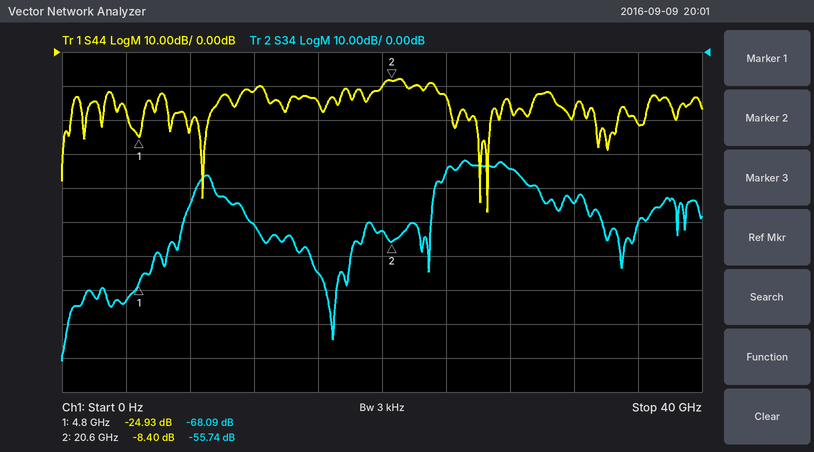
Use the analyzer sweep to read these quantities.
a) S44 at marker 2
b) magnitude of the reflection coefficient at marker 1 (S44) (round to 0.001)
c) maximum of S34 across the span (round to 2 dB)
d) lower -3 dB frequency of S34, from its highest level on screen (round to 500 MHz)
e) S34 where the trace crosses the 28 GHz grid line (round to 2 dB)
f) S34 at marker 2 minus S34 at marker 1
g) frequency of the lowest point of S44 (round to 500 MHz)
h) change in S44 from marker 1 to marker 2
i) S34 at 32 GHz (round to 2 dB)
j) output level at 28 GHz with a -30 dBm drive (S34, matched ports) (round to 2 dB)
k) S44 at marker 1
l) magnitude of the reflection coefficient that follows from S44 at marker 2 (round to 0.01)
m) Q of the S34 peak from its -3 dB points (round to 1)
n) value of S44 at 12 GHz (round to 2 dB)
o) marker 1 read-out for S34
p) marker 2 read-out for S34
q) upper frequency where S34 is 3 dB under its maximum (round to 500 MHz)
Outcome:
-8.40 dB
0.057
-32 dB
24.0 GHz
-34 dB
12.35 dB
26.5 GHz
16.53 dB
-44 dB
-64 dBm
-24.93 dB
0.38
6
-12 dB
-68.09 dB
-55.74 dB
28.5 GHz
